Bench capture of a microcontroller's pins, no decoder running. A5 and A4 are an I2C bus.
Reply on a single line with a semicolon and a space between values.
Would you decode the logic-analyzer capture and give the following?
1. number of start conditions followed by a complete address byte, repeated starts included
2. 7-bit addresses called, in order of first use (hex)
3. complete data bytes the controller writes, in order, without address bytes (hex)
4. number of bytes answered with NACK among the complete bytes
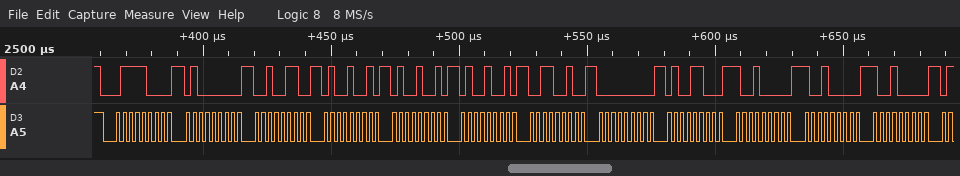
1; 0x3C; 40 26 49 49 49 32 00 4C 90 90 90; 0
